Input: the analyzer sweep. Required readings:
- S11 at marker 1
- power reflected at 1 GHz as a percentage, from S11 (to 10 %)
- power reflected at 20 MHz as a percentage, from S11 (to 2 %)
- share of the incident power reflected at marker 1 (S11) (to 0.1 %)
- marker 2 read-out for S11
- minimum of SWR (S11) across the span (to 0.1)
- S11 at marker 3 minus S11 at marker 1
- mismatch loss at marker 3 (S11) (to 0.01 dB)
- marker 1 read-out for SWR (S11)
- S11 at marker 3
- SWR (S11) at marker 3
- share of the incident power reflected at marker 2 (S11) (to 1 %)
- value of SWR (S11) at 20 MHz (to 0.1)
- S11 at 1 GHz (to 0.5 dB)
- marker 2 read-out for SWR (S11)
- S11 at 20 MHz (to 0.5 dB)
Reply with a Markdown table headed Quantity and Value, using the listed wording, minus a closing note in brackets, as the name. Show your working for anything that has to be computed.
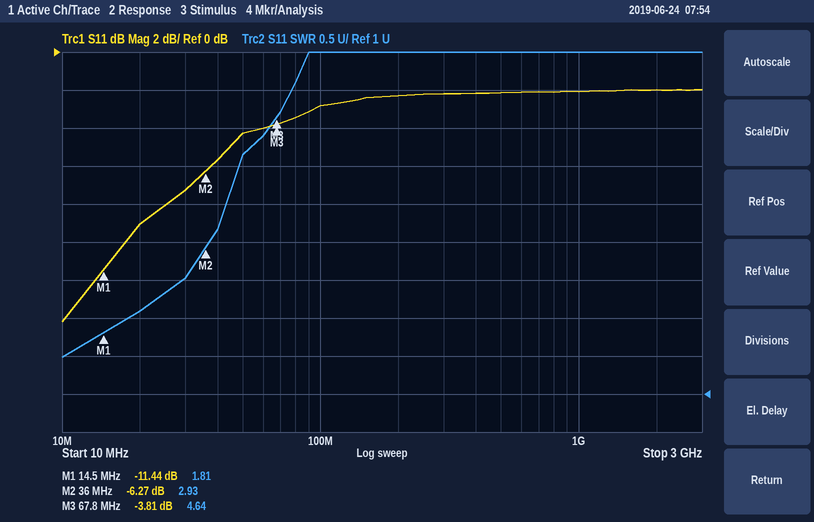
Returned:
| Quantity | Value |
|---|---|
| S11 at marker 1 | -11.44 dB |
| power reflected at 1 GHz as a percentage, from S11 | 10^(-2/10) ≈ 63.1 %, so 60 % to the nearest 10 % |
| power reflected at 20 MHz as a percentage, from S11 | 10^(-9/10) ≈ 12.6 %, so 12 % to the nearest 2 % |
| share of the incident power reflected at marker 1 (S11) | 10^(-11.44/10) ≈ 7.2 % |
| marker 2 read-out for S11 | -6.27 dB |
| minimum of SWR (S11) across the span | 1.5 |
| S11 at marker 3 minus S11 at marker 1 | -3.81 − (-11.44) = 7.63 dB |
| mismatch loss at marker 3 (S11) | −10 log10(1 − 10^(-3.81/10)) ≈ 2.34 dB |
| marker 1 read-out for SWR | 1.81 |
| S11 at marker 3 | -3.81 dB |
| SWR (S11) at marker 3 | 4.64 |
| share of the incident power reflected at marker 2 (S11) | 10^(-6.27/10) ≈ 24 % |
| value of SWR (S11) at 20 MHz | 2.1 |
| S11 at 1 GHz | -2.0 dB |
| marker 2 read-out for SWR | 2.93 |
| S11 at 20 MHz | -9.0 dB |
